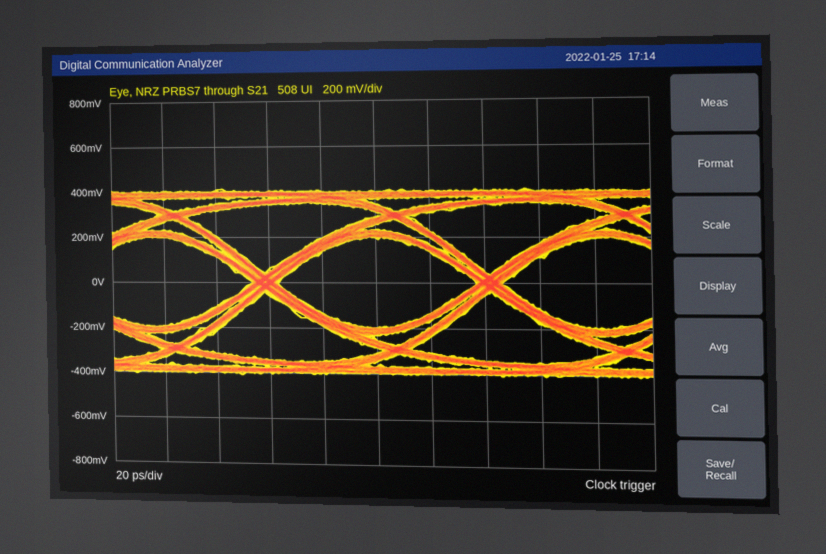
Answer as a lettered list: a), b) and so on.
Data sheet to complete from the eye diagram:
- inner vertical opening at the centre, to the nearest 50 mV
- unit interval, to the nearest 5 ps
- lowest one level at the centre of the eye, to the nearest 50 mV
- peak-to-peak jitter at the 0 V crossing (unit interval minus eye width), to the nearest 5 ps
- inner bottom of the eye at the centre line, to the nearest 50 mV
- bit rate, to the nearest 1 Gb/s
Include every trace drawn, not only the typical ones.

a) 400 mV
b) 85 ps
c) 200 mV
d) 10 ps
e) -200 mV
f) 12 Gb/s
